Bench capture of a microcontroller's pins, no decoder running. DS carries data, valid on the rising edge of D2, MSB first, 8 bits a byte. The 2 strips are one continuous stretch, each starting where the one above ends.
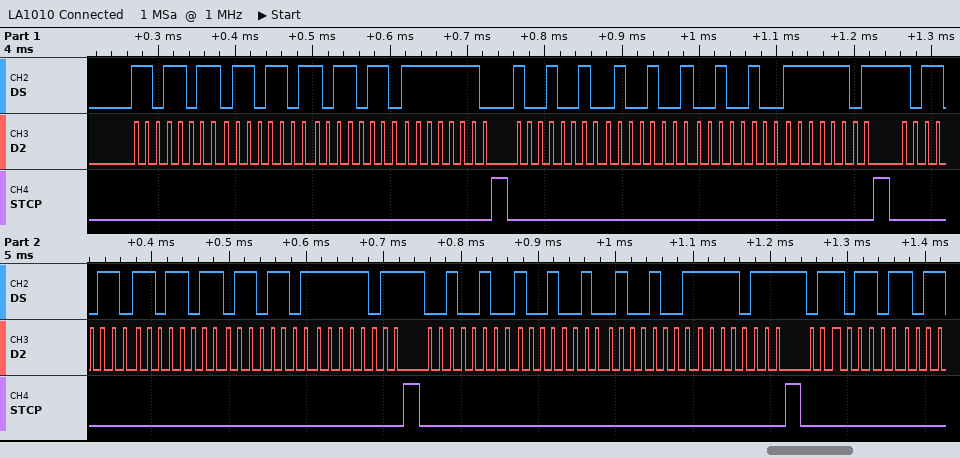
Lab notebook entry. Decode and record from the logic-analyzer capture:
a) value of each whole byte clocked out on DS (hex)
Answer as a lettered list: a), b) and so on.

a) DB 6D B6 FE 92 49 24 FD B6 DB 6D FB 24 92 49 F7 6D
